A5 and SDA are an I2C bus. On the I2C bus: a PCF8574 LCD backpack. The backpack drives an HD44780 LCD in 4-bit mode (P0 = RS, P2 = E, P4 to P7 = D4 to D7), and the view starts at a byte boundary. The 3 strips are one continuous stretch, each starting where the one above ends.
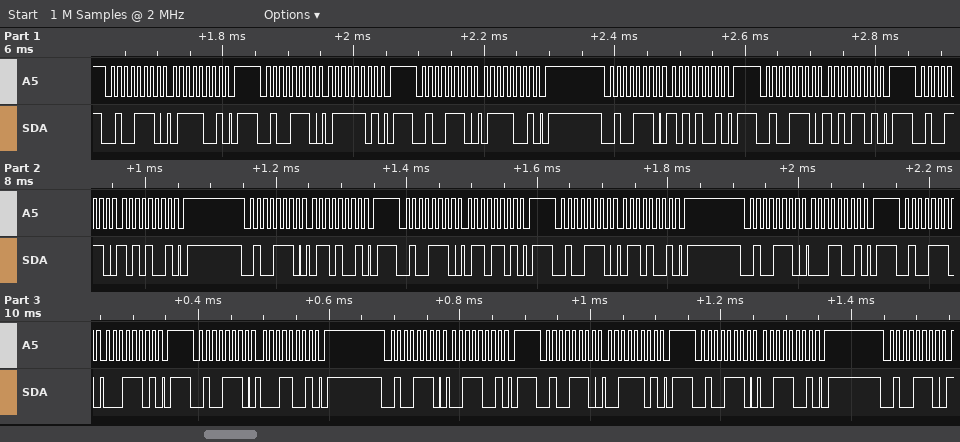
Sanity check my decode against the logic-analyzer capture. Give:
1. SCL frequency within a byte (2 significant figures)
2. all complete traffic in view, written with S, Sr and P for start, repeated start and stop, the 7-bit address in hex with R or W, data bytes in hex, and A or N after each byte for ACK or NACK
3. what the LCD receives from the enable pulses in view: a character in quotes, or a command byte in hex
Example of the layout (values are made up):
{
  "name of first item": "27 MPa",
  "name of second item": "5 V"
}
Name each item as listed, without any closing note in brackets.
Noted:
{
  "SCL frequency within a byte": "100 kHz",
  "all complete traffic in view, written with S, Sr and P for start, repeated start and stop, the 7-bit address in hex with R or W, data bytes in hex, and A or N after each byte for ACK or NACK": "S 27W A 79 A P S 27W A 7D A P S 27W A 79 A P S 27W A A9 A P S 27W A AD A P S 27W A A9 A P S 27W A 69 A P S 27W A 6D A P S 27W A 69 A P S 27W A 19 A P S 27W A 1D A P S 27W A 19 A P S 27W A 39 A P S 27W A 3D A P S 27W A 39 A P S 27W A",
  "what the LCD receives from the enable pulses in view: a character in quotes, or a command byte in hex": "'z' 'a'"
}
